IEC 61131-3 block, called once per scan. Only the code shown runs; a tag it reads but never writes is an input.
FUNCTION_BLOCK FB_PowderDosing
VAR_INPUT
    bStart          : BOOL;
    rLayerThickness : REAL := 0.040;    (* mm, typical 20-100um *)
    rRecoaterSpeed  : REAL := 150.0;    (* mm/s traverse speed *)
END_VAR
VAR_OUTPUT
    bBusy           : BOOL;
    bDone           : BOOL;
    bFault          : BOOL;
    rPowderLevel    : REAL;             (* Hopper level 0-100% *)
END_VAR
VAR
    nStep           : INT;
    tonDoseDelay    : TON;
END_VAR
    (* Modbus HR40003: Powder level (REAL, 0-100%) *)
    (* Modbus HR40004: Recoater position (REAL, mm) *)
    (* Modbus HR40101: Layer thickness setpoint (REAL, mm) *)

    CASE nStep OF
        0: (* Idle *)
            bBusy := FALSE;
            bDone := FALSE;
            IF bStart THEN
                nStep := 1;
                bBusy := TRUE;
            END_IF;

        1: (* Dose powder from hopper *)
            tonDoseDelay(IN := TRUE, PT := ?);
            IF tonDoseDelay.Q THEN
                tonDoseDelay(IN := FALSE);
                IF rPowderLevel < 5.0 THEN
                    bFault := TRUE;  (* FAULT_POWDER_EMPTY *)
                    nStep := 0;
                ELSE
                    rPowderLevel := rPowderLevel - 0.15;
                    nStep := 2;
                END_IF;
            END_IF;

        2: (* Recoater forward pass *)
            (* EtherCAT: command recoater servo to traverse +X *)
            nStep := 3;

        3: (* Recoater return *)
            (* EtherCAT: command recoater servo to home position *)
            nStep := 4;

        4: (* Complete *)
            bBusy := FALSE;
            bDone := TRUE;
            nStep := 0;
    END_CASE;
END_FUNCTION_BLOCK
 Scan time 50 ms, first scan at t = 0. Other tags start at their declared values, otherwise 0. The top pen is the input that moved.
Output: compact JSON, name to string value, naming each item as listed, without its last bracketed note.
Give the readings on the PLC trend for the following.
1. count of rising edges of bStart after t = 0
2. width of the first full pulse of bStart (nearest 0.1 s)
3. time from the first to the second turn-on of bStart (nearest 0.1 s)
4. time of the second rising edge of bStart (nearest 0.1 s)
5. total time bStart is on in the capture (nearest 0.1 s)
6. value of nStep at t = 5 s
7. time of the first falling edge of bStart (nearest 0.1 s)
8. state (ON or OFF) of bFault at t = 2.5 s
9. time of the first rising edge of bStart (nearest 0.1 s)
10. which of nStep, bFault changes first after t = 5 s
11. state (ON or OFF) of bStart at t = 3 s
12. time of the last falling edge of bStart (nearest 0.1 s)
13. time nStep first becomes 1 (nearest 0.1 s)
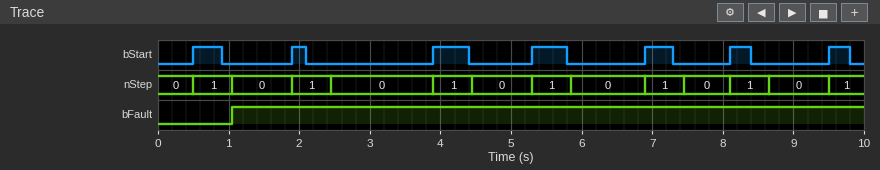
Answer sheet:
{"count of rising edges of bStart after t = 0": "7", "width of the first full pulse of bStart": "0.4 s", "time from the first to the second turn-on of bStart": "1.4 s", "time of the second rising edge of bStart": "1.9 s", "total time bStart is on in the capture": "2.6 s", "value of nStep at t = 5 s": "0", "time of the first falling edge of bStart": "0.9 s", "state (ON or OFF) of bFault at t = 2.5 s": "ON", "time of the first rising edge of bStart": "0.5 s", "which of nStep, bFault changes first after t = 5 s": "nStep", "state (ON or OFF) of bStart at t = 3 s": "OFF", "time of the last falling edge of bStart": "9.8 s", "time nStep first becomes 1": "0.5 s"}
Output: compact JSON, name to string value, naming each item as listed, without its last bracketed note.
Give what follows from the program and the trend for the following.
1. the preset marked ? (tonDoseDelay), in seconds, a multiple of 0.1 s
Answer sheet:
{"the preset marked ? (tonDoseDelay), in seconds, a multiple of 0.1 s": "0.5 s"}
